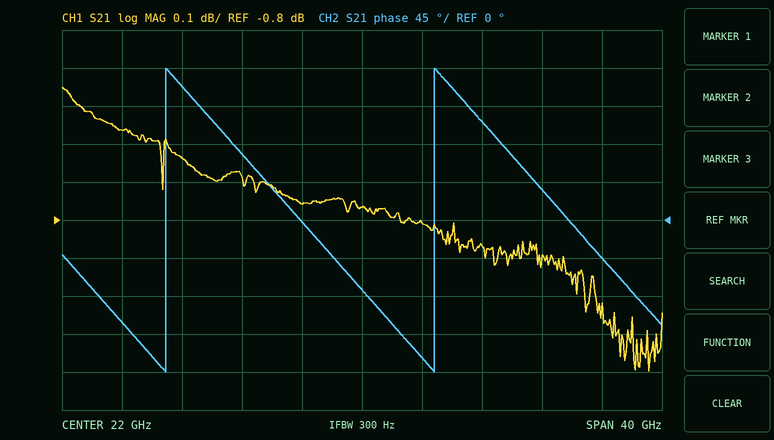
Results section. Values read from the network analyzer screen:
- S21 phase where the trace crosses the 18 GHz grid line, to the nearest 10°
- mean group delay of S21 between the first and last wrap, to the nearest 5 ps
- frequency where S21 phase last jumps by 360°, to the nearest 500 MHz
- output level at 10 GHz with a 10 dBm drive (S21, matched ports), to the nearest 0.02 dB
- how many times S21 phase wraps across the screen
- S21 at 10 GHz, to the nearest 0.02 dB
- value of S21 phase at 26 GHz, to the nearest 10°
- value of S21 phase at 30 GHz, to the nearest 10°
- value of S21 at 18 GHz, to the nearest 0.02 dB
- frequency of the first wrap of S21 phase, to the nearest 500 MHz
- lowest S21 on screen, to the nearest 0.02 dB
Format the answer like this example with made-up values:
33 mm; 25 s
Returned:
0°; 55 ps; 27.0 GHz; 9.36 dBm; 2; -0.64 dB; -160°; 120°; -0.76 dB; 9.0 GHz; -1.20 dB
